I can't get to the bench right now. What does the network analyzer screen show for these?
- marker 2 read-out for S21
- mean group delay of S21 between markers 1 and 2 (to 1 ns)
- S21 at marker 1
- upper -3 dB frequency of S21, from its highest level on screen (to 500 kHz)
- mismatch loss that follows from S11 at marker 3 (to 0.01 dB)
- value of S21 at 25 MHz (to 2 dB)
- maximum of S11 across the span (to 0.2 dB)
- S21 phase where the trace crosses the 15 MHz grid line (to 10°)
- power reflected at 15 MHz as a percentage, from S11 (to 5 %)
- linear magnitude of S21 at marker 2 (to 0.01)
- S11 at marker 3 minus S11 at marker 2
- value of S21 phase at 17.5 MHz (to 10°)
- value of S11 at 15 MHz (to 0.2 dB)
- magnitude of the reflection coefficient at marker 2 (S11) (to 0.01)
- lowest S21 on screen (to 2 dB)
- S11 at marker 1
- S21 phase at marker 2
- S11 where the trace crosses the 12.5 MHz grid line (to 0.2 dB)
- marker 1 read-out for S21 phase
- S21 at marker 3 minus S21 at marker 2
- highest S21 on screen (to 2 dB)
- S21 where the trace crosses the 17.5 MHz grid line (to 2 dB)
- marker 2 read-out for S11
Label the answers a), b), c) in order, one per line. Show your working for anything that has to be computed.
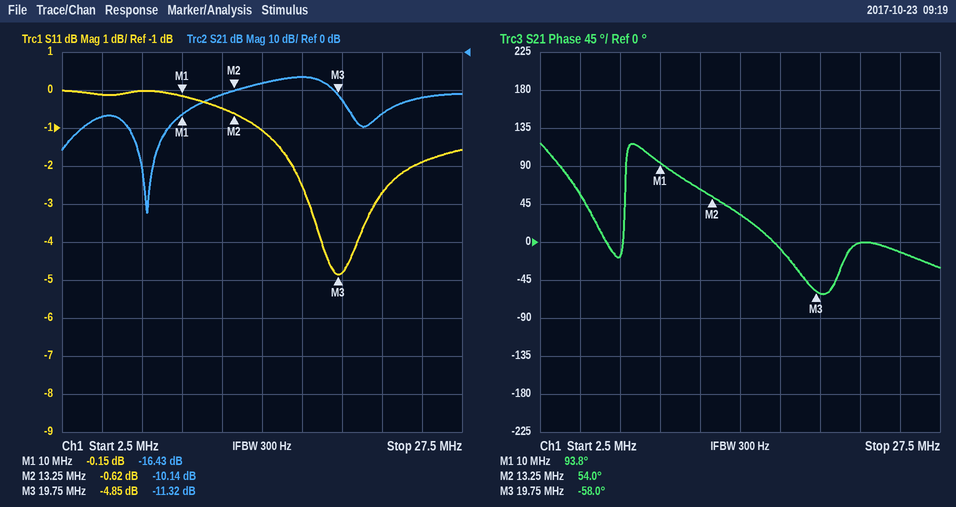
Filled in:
a) -10.14 dB
b) −(54° − (93.8°))/(360° × 3.25 MHz) ≈ 34 ns
c) -16.43 dB
d) 19.5 MHz
e) −10 log10(1 − 10^(-4.85/10)) ≈ 1.72 dB
f) -12 dB
g) 0.0 dB
h) 30°
i) 10^(-1/10) ≈ 79.4 %, so 80 % to the nearest 5 %
j) 10^(-10.14/20) ≈ 0.31
k) -4.85 − (-0.62) = -4.23 dB
l) -10°
m) -1.0 dB
n) 10^(-0.62/20) ≈ 0.93
o) -42 dB
p) -0.15 dB
q) 54.0°
r) -0.4 dB
s) 93.8°
t) -11.32 − (-10.14) = -1.18 dB
u) -6 dB
v) -6 dB
w) -0.62 dB
